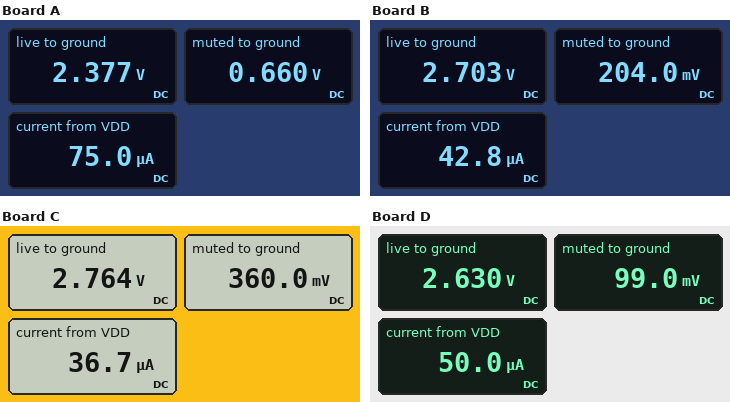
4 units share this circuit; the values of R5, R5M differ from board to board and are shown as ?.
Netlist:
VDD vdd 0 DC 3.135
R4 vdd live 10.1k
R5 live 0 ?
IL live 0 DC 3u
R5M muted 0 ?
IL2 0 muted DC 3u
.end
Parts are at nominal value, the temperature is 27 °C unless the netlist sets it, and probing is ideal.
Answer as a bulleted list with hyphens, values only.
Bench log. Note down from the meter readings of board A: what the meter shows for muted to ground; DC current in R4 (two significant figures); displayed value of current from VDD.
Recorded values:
- 0.660 V
- 75 µA
- 75.0 µA
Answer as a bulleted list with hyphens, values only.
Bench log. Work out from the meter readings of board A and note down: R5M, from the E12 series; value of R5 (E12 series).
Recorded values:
- 220 kΩ
- 33 kΩ
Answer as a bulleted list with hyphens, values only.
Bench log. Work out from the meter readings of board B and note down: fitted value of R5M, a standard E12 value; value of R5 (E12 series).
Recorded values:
- 68 kΩ
- 68 kΩ
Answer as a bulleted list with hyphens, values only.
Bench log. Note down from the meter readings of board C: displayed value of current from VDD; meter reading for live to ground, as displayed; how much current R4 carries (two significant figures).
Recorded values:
- 36.7 µA
- 2.764 V
- 37 µA
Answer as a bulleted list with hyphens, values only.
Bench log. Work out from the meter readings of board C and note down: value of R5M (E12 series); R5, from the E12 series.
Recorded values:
- 120 kΩ
- 82 kΩ
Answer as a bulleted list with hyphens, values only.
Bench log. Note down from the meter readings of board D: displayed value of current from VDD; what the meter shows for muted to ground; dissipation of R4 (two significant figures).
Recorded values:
- 50.0 µA
- 99.0 mV
- 25 µW
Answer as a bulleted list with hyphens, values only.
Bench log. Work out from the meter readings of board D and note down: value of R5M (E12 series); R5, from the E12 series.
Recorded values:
- 33 kΩ
- 56 kΩ
